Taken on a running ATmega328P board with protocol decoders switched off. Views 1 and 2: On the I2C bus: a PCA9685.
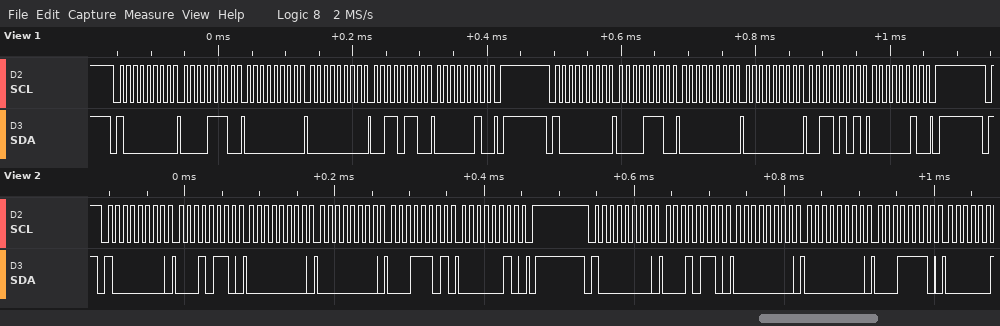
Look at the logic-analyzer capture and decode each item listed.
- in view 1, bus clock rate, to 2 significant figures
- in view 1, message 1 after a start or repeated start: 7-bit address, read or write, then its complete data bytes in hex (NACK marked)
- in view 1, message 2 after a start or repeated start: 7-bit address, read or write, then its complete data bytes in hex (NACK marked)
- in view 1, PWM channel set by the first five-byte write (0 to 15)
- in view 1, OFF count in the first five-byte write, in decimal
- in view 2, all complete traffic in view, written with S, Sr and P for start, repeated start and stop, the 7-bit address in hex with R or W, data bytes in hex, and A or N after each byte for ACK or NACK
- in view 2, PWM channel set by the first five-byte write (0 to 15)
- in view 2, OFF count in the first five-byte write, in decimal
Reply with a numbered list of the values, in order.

1. 100 kHz
2. 0x40 write: 0E 00 00 36 02
3. 0x40 write: 0E 00 00 35 02
4. 2
5. 566
6. S 40W A 16 A 00 A 00 A 1D A 02 A P S 40W A 16 A 00 A 00 A 1E A
7. 4
8. 541
